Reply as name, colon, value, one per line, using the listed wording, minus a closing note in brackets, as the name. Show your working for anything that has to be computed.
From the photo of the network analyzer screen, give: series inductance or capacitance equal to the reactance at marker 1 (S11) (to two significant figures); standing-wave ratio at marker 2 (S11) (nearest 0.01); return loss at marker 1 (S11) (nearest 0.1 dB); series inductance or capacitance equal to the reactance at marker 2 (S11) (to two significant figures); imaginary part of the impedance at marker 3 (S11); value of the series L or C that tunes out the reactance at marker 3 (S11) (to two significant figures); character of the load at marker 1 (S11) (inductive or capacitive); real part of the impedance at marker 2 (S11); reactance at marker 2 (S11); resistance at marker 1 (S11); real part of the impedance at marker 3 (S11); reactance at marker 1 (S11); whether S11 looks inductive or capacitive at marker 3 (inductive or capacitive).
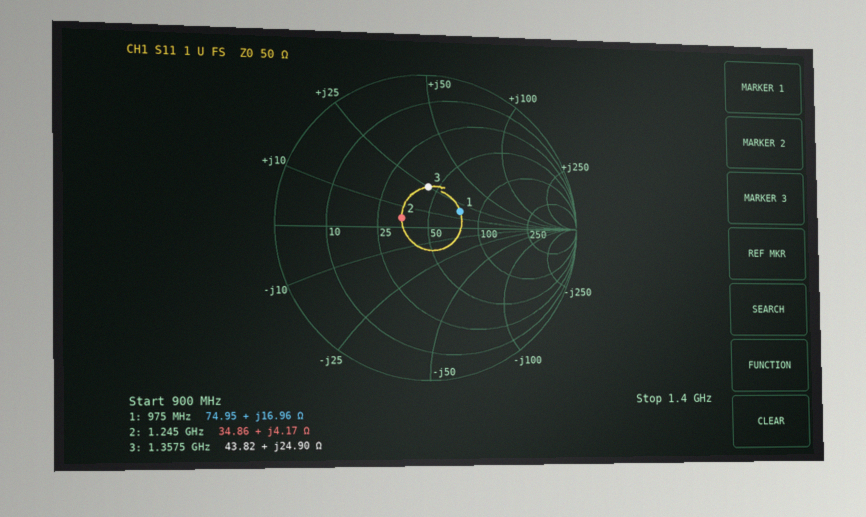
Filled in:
series inductance or capacitance equal to the reactance at marker 1 (S11): L = 16.96 Ω/(2π × 975 MHz) ≈ 2.8 nH
standing-wave ratio at marker 2 (S11): 1.45
return loss at marker 1 (S11): 12.4 dB
series inductance or capacitance equal to the reactance at marker 2 (S11): L = 4.17 Ω/(2π × 1.245 GHz) ≈ 533 pH, so 530 pH to two significant figures
imaginary part of the impedance at marker 3: +24.90 Ω
value of the series L or C that tunes out the reactance at marker 3 (S11): C = 1/(2π × 1.3575 GHz × 24.9 Ω) ≈ 4.7 pF
character of the load at marker 1 (S11): inductive
real part of the impedance at marker 2: 34.86 Ω
reactance at marker 2: +4.17 Ω
resistance at marker 1: 74.95 Ω
real part of the impedance at marker 3: 43.82 Ω
reactance at marker 1: +16.96 Ω
whether S11 looks inductive or capacitive at marker 3: inductive
